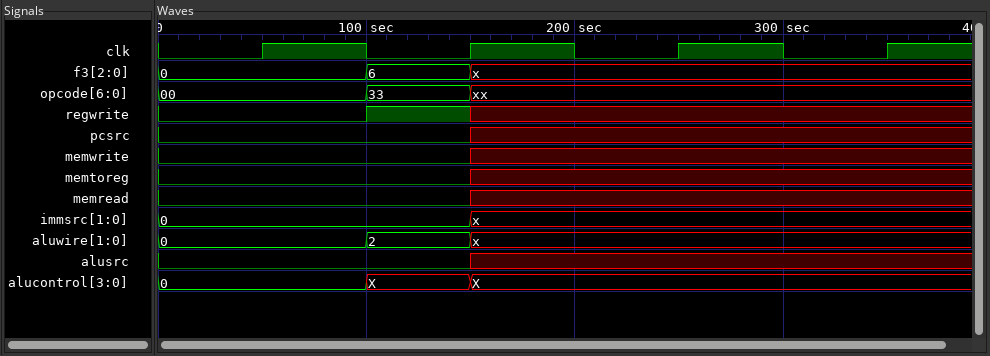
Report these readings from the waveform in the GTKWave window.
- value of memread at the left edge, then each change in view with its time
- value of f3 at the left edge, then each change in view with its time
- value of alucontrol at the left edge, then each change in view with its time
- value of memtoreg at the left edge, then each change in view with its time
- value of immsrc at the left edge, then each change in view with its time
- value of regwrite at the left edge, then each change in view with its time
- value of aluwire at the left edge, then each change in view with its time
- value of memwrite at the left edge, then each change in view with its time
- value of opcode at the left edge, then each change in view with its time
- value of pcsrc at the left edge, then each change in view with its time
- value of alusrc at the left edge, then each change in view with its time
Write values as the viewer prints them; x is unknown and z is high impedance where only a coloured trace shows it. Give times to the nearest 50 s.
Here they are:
0, x at 150 s
0, 6 at 100 s, x at 150 s
0, X at 100 s, X at 150 s
0, x at 150 s
0, x at 150 s
0, 1 at 100 s, x at 150 s
0, 2 at 100 s, x at 150 s
0, x at 150 s
00, 33 at 100 s, xx at 150 s
0, x at 150 s
0, x at 150 s
